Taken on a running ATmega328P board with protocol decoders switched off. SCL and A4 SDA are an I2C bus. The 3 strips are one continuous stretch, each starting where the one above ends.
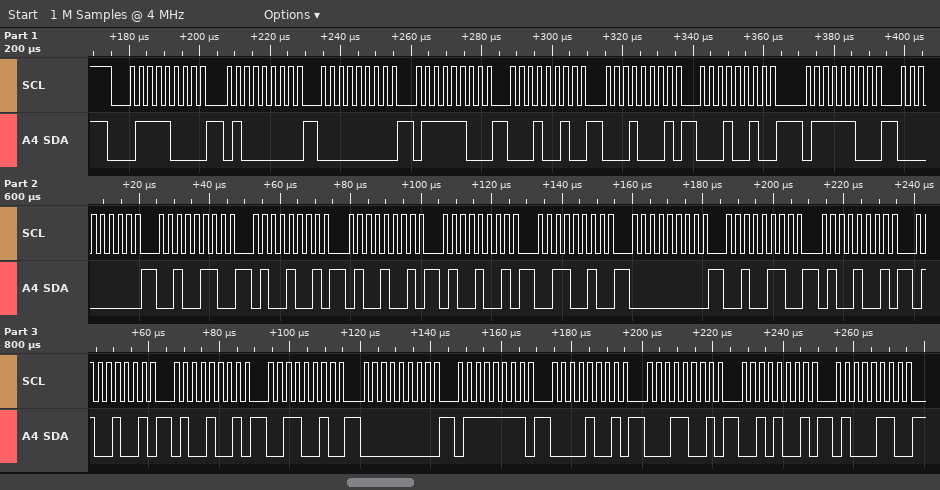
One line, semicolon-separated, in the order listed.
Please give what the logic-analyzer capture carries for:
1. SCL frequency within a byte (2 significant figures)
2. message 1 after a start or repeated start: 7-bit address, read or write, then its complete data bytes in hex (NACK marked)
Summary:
400 kHz; 0x3C write: 40 00 7C 12 11 12 7C 00 26 49 49 49 32 00 26 49 49 49 32 00 7F 09 19 29 46
